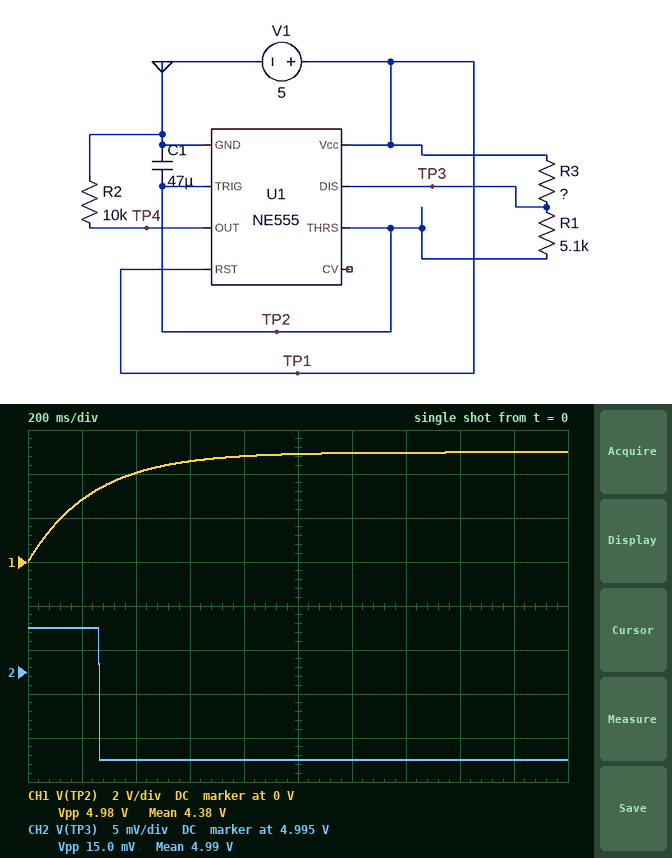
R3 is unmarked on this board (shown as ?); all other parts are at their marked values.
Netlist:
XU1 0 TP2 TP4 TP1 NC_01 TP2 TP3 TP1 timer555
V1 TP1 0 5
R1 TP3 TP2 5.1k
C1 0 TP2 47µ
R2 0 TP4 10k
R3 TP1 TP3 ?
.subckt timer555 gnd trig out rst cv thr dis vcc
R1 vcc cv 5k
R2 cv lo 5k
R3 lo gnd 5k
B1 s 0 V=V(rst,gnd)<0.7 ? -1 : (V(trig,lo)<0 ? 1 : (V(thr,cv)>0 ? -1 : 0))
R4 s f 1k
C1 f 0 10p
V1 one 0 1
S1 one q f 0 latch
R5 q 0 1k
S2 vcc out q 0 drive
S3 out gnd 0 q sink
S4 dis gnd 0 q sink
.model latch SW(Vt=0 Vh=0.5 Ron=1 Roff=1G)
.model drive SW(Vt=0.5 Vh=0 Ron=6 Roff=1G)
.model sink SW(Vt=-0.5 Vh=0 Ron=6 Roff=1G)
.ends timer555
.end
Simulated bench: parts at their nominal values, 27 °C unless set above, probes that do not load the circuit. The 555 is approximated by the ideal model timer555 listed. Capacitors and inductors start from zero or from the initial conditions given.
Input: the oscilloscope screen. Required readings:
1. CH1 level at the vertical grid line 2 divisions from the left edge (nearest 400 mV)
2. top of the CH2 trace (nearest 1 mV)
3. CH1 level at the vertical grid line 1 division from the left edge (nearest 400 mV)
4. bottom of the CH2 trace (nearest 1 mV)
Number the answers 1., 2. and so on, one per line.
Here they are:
1. 4.0 V
2. 5.000 V
3. 2.8 V
4. 4.985 V
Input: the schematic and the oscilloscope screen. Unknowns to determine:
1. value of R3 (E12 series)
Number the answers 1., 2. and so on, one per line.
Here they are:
1. 0.018 Ω
